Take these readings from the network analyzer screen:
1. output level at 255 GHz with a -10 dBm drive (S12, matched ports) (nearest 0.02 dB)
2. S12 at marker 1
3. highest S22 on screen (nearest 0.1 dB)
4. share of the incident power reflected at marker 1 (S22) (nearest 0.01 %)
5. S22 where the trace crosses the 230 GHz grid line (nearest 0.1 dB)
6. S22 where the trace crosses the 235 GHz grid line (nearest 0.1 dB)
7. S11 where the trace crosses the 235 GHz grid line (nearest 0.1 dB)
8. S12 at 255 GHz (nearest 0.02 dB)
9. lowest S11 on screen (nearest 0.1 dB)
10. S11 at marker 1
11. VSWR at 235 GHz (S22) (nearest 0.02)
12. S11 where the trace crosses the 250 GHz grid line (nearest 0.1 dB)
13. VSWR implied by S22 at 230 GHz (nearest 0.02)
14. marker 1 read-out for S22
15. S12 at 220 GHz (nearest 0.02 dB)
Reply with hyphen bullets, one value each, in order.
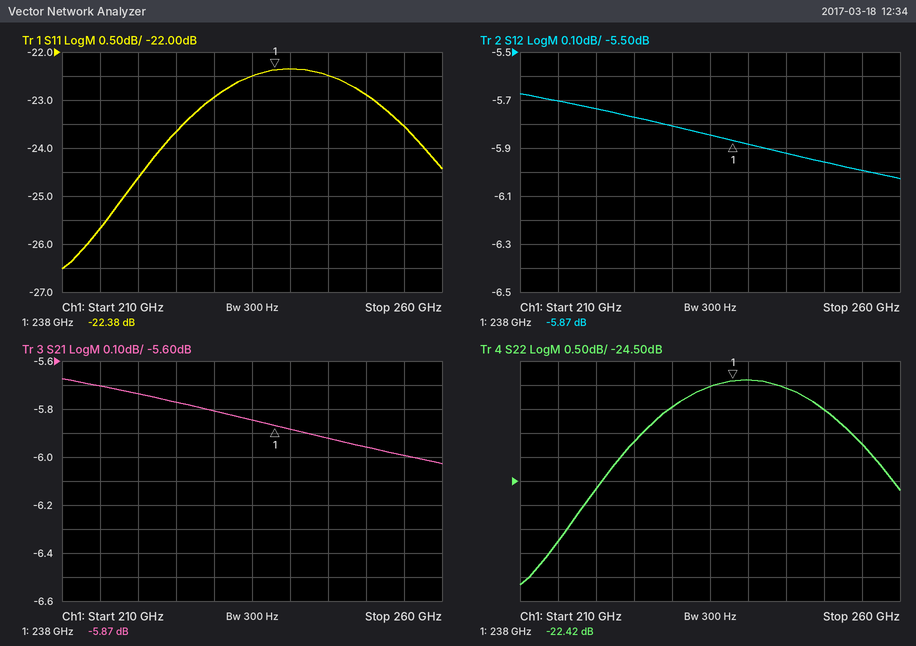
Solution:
- -16.00 dBm
- -5.87 dB
- -22.4 dB
- 0.57 %
- -23.0 dB
- -22.5 dB
- -22.5 dB
- -6.00 dB
- -26.5 dB
- -22.38 dB
- 1.16
- -22.9 dB
- 1.16
- -22.42 dB
- -5.74 dB
